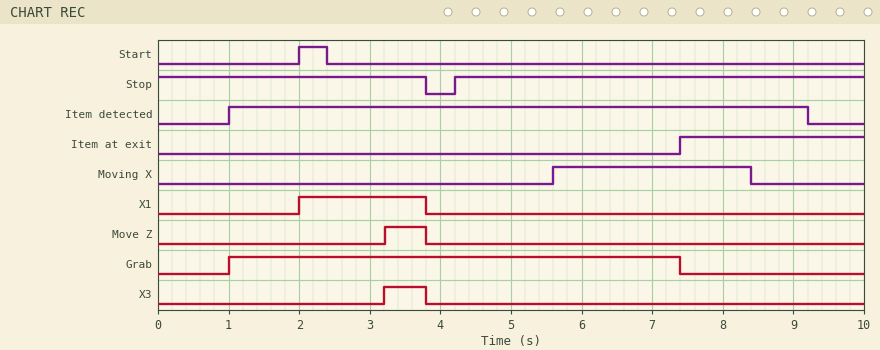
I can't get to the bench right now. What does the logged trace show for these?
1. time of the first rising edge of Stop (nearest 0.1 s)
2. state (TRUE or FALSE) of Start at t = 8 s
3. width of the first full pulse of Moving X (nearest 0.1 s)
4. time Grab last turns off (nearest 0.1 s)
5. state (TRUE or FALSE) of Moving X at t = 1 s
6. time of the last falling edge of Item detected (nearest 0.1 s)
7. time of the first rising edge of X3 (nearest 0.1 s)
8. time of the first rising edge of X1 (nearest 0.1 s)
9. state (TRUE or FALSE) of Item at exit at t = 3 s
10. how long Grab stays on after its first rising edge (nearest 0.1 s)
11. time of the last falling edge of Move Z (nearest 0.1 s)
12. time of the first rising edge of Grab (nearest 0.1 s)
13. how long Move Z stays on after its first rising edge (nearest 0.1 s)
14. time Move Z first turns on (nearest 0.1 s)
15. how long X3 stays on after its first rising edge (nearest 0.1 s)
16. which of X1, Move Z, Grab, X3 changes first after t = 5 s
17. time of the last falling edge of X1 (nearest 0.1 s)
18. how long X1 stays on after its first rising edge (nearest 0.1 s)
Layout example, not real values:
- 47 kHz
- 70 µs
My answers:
- 4.2 s
- FALSE
- 2.8 s
- 7.4 s
- FALSE
- 9.2 s
- 3.2 s
- 2.0 s
- FALSE
- 6.4 s
- 3.8 s
- 1.0 s
- 0.6 s
- 3.2 s
- 0.6 s
- Grab
- 3.8 s
- 1.8 s
